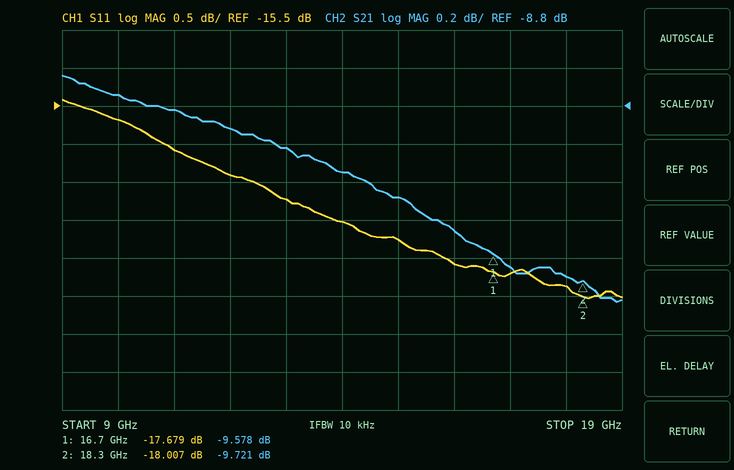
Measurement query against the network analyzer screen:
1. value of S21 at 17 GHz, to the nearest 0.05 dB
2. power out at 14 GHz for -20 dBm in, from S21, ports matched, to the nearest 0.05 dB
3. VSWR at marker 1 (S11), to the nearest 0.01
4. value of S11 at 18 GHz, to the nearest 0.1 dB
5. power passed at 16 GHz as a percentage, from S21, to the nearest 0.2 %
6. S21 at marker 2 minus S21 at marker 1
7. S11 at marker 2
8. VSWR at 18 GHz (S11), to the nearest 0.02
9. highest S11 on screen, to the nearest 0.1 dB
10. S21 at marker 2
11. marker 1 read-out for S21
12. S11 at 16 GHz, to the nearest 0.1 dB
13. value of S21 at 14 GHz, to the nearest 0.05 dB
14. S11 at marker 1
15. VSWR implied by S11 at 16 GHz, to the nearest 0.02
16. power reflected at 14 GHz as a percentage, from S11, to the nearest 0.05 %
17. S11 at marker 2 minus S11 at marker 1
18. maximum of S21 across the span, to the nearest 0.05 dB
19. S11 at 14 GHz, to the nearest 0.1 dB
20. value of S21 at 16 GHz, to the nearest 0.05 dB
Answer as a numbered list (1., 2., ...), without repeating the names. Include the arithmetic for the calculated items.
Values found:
1. -9.65 dB
2. -20 dBm + (-9.15 dB) = -29.15 dBm
3. (1 + 0.1306)/(1 − 0.1306) ≈ 1.30
4. -17.9 dB
5. 10^(-9.45/10) ≈ 11.4 %
6. -9.721 − (-9.578) = -0.143 dB
7. -18.007 dB
8. |Γ| = 10^(-17.9/20) = 0.1274; VSWR = (1 + 0.1274)/(1 − 0.1274) ≈ 1.29, so 1.30 to the nearest 0.02
9. -15.4 dB
10. -9.721 dB
11. -9.578 dB
12. -17.6 dB
13. -9.15 dB
14. -17.679 dB
15. |Γ| = 10^(-17.6/20) = 0.1318; VSWR = (1 + 0.1318)/(1 − 0.1318) ≈ 1.30
16. 10^(-17/10) ≈ 2.00 %
17. -18.007 − (-17.679) = -0.328 dB
18. -8.65 dB
19. -17.0 dB
20. -9.45 dB
